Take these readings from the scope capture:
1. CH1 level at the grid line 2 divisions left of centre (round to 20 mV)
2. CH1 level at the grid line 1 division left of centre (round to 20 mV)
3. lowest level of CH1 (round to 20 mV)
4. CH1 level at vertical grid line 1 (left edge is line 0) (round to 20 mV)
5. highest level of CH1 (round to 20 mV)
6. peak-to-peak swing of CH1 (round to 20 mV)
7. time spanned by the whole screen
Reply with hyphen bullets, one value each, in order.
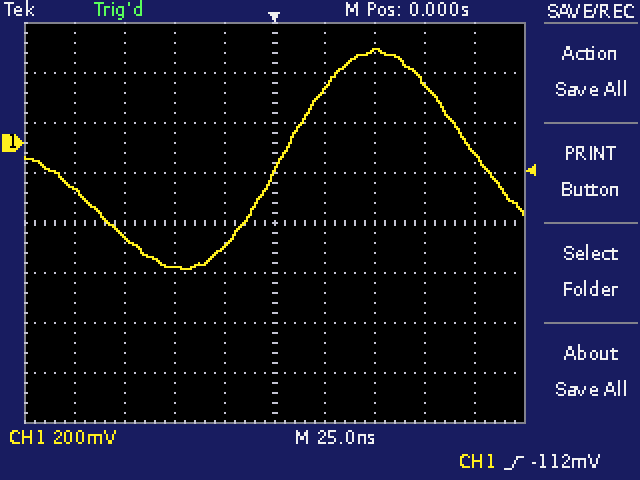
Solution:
- -500 mV
- -420 mV
- -500 mV
- -180 mV
- 380 mV
- 880 mV
- 250 ns
